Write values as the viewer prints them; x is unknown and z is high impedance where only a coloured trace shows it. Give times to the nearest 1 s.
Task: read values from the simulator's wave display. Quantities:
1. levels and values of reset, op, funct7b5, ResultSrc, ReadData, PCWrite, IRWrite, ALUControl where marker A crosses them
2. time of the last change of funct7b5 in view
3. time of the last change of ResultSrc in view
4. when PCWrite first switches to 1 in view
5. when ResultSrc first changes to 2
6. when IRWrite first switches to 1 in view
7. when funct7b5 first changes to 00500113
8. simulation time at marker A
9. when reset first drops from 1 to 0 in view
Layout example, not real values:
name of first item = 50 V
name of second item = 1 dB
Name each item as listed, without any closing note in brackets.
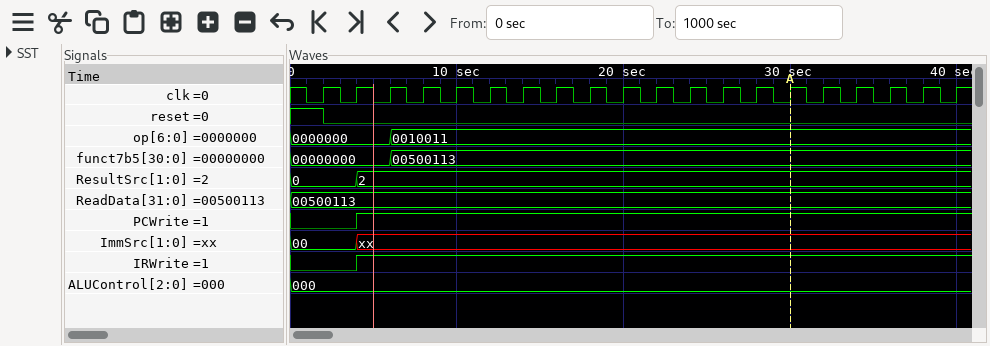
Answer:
levels and values of reset, op, funct7b5, ResultSrc, ReadData, PCWrite, IRWrite, ALUControl where marker A crosses them = reset=0, op=0010011, funct7b5=00500113, ResultSrc=2, ReadData=00500113, PCWrite=1, IRWrite=1, ALUControl=000
time of the last change of funct7b5 in view = 6 s
time of the last change of ResultSrc in view = 4 s
when PCWrite first switches to 1 in view = 4 s
when ResultSrc first changes to 2 = 4 s
when IRWrite first switches to 1 in view = 4 s
when funct7b5 first changes to 00500113 = 6 s
simulation time at marker A = 30 s
when reset first drops from 1 to 0 in view = 2 s
